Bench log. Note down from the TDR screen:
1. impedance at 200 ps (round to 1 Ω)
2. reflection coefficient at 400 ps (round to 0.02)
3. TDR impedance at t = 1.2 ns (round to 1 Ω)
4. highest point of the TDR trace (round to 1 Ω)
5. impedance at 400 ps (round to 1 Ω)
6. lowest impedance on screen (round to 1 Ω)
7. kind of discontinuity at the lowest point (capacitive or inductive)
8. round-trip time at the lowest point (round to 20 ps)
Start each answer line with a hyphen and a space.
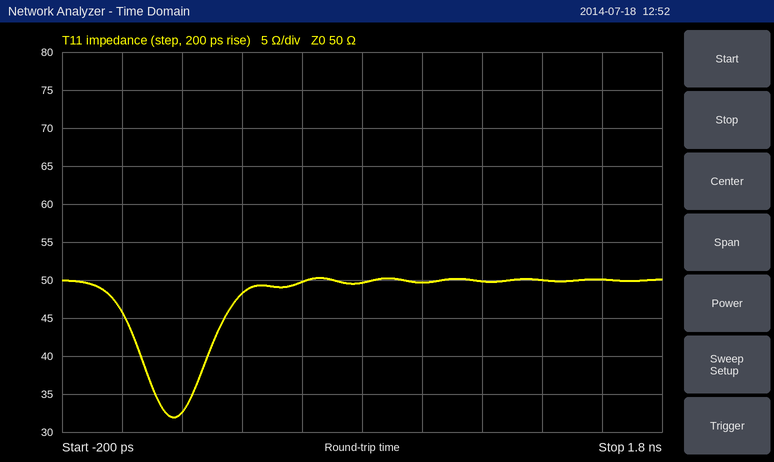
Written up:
- 33 Ω
- -0.02
- 50 Ω
- 50 Ω
- 48 Ω
- 32 Ω
- capacitive
- 180 ps
